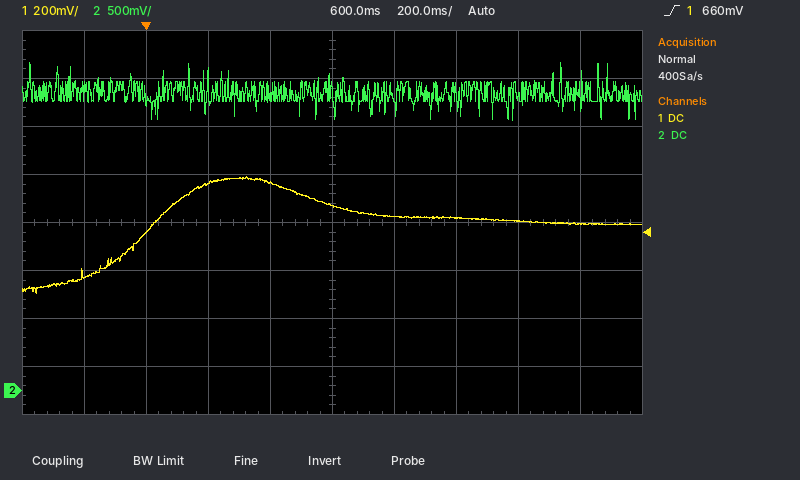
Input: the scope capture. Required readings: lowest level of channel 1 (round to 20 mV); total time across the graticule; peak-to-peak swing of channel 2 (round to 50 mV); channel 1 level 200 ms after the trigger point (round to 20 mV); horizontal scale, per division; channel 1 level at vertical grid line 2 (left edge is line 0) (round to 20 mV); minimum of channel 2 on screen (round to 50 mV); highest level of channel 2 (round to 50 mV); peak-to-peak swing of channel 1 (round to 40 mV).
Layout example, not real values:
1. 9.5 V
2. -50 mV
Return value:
1. 400 mV
2. 2 s
3. 600 mV
4. 860 mV
5. 200 ms
6. 660 mV
7. 2.80 V
8. 3.40 V
9. 480 mV
